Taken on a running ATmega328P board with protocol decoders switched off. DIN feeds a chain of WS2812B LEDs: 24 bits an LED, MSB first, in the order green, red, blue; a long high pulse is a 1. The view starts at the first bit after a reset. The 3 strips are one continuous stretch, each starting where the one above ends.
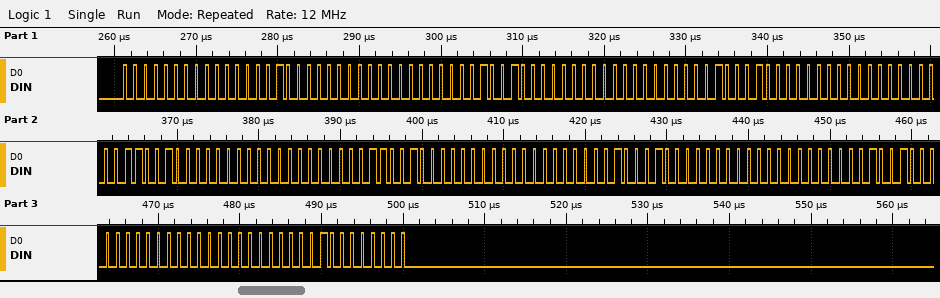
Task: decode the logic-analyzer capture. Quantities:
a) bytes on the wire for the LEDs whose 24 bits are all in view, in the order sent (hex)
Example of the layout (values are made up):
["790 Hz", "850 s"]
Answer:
["00 01 00 00 12 00 00 22 00 00 32 00 00 32 00 00 22 00 00 12 00 00 01 00"]
